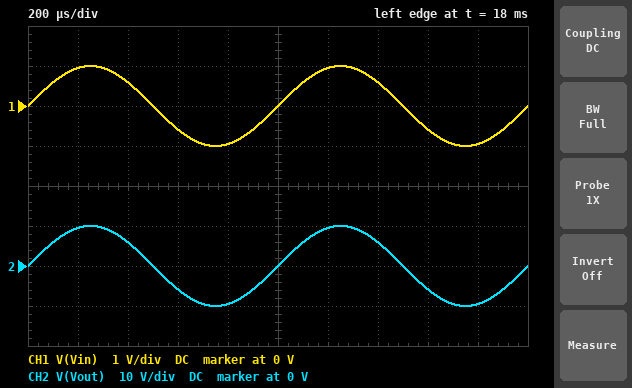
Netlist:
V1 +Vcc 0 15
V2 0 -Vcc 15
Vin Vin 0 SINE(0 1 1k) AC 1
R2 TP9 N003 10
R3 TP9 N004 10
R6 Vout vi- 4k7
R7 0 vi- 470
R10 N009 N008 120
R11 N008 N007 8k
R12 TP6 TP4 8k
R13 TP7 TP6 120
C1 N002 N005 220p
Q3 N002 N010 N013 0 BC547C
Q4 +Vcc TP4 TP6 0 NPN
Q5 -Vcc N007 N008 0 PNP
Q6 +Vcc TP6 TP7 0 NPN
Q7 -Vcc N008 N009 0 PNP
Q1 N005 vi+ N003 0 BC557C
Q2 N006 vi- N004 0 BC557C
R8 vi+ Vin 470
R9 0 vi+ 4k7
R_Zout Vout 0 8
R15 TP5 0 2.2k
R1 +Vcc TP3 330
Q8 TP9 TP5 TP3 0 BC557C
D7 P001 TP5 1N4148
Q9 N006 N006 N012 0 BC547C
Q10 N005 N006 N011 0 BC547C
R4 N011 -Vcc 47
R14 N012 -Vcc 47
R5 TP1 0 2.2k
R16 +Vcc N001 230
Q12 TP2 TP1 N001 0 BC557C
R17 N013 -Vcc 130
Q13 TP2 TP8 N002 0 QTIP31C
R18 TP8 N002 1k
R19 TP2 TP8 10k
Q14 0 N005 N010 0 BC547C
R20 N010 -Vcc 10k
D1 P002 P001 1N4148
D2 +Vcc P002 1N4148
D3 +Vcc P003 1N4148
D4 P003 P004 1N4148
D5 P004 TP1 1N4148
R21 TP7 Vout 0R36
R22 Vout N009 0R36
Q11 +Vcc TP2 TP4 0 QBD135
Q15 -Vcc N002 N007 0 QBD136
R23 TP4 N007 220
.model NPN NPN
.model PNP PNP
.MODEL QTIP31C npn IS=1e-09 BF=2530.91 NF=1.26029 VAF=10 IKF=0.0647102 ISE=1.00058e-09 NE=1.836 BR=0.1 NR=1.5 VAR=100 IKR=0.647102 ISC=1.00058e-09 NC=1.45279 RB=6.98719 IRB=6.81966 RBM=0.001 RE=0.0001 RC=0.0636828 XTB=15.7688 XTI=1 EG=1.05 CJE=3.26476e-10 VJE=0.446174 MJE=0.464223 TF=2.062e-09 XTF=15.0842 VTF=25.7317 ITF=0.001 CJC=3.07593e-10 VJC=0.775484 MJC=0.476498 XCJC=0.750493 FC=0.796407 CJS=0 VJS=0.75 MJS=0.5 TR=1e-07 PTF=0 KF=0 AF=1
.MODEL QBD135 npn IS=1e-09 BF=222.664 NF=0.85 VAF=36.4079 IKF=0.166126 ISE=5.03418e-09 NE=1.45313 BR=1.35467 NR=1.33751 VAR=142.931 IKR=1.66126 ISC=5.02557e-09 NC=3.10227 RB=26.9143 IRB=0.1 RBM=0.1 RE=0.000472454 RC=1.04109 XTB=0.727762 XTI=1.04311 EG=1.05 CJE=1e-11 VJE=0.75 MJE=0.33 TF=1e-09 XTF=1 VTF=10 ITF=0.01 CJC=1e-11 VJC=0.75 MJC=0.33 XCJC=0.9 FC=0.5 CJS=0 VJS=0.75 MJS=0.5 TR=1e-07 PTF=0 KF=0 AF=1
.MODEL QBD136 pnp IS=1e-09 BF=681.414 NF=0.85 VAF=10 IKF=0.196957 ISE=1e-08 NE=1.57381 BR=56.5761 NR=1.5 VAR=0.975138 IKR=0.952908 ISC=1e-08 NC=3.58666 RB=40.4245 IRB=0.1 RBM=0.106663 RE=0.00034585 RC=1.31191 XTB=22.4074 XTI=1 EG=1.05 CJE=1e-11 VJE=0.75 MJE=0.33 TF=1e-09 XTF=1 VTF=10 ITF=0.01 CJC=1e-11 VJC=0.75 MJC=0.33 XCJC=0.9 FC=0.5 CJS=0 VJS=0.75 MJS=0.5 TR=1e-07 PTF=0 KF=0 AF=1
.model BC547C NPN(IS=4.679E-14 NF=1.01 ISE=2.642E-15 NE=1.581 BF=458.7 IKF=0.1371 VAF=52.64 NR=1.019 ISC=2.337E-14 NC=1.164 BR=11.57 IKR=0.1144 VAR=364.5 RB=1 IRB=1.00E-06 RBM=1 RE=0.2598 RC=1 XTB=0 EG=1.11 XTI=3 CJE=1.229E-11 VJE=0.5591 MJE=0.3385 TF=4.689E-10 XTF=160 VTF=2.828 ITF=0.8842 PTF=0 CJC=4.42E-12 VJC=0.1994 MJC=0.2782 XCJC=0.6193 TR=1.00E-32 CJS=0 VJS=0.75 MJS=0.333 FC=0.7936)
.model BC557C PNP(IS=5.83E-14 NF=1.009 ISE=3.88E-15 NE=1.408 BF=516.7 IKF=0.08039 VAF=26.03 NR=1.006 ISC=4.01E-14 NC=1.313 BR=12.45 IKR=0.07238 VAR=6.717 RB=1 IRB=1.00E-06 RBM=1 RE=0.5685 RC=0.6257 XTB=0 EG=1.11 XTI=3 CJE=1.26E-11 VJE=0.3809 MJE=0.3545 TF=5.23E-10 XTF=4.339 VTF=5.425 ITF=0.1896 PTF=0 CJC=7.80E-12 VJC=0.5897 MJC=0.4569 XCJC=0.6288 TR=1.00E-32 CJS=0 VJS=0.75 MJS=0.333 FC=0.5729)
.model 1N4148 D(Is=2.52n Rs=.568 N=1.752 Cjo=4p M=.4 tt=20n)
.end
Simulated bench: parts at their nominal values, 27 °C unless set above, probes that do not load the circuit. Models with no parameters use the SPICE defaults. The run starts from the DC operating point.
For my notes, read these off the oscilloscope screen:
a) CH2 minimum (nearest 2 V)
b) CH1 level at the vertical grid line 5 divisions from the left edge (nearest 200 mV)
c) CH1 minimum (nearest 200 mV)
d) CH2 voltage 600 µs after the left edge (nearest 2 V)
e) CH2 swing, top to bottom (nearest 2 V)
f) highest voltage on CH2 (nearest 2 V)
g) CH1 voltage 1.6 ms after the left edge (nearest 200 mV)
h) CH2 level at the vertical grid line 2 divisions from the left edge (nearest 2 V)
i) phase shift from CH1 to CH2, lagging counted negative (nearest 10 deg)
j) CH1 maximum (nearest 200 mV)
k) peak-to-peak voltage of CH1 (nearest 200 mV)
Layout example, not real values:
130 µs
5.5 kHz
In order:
-10 V
0 V
-1.0 V
-6 V
20 V
10 V
-600 mV
6 V
0 deg
1.0 V
2.0 V
